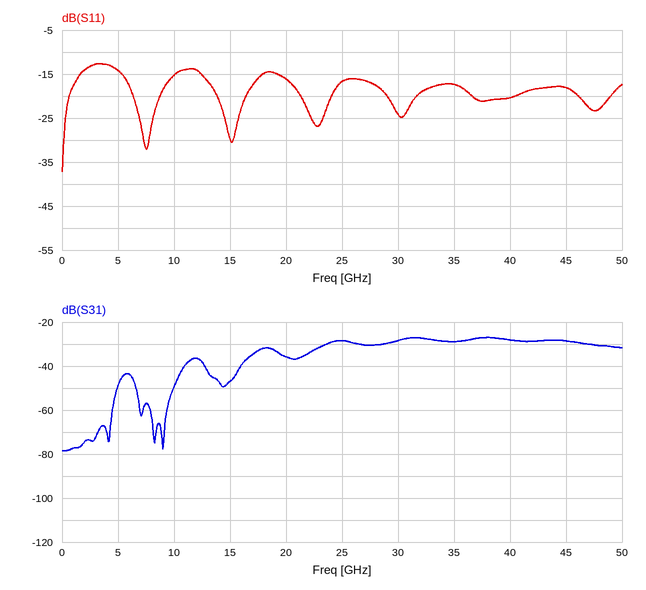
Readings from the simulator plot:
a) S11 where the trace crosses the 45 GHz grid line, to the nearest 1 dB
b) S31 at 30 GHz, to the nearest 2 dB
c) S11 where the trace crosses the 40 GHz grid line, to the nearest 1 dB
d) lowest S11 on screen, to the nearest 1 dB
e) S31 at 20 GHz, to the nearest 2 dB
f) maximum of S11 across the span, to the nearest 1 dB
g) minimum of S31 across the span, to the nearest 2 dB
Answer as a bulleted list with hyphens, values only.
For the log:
- -18 dB
- -28 dB
- -20 dB
- -37 dB
- -36 dB
- -13 dB
- -78 dB
